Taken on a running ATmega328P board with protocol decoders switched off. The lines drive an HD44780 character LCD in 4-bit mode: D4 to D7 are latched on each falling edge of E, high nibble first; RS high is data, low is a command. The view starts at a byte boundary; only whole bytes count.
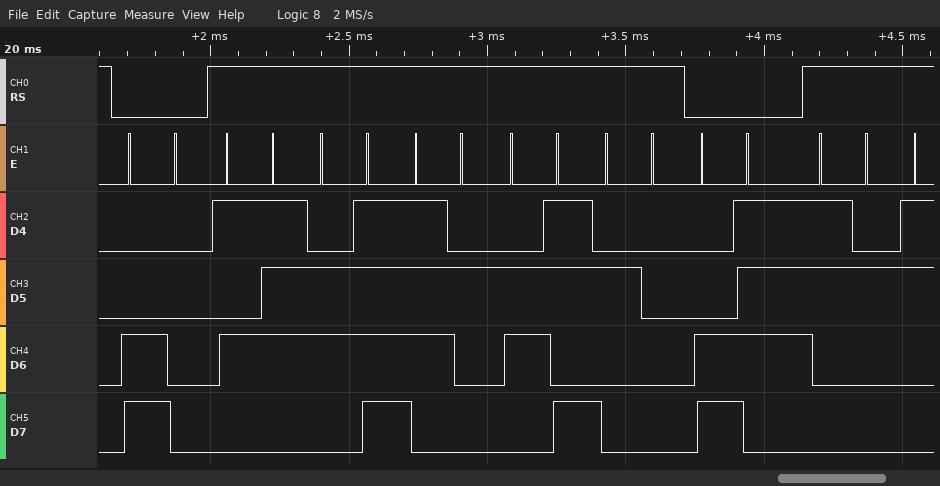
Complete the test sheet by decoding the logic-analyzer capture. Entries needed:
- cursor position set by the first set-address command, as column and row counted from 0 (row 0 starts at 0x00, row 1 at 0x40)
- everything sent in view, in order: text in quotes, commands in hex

column 0, row 1
0xC0 "Work " 0xC7 "2"
